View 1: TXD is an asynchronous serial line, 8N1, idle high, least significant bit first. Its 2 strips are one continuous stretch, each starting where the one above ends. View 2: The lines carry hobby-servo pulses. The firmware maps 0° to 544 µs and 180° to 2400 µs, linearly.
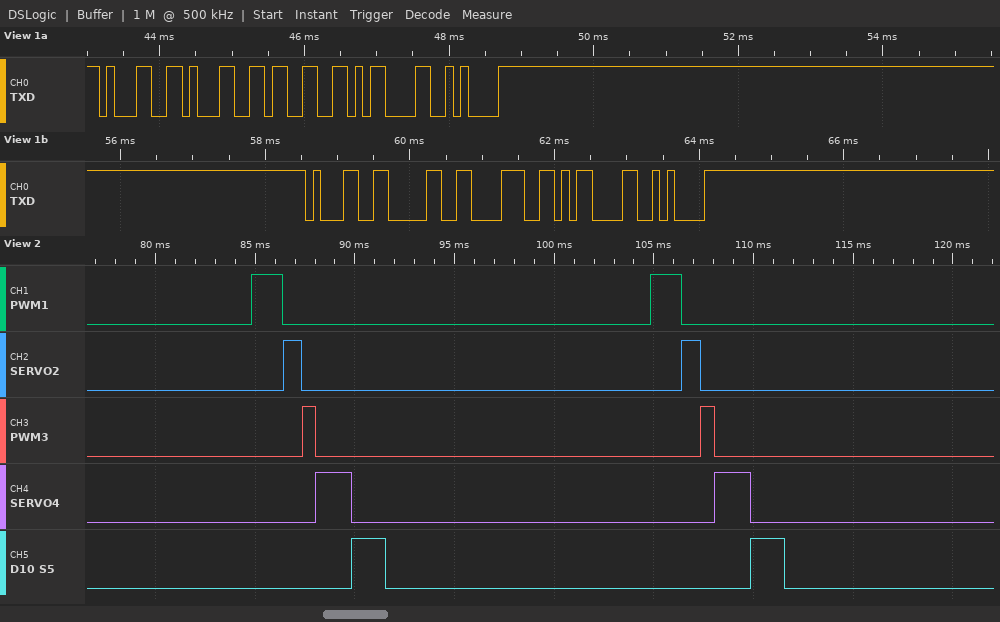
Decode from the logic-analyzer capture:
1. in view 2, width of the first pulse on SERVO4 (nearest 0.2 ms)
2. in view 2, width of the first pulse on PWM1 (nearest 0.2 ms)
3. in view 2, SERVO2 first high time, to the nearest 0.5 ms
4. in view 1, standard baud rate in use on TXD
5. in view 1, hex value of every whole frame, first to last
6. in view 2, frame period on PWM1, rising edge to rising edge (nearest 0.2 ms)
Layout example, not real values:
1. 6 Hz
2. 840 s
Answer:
1. 1.8 ms
2. 1.6 ms
3. 1.0 ms
4. 9600 baud
5. 0x31 0x31 0x33 0x0D 0x0A 0x31 0x30 0x38 0x0D 0x0A
6. 20.0 ms
